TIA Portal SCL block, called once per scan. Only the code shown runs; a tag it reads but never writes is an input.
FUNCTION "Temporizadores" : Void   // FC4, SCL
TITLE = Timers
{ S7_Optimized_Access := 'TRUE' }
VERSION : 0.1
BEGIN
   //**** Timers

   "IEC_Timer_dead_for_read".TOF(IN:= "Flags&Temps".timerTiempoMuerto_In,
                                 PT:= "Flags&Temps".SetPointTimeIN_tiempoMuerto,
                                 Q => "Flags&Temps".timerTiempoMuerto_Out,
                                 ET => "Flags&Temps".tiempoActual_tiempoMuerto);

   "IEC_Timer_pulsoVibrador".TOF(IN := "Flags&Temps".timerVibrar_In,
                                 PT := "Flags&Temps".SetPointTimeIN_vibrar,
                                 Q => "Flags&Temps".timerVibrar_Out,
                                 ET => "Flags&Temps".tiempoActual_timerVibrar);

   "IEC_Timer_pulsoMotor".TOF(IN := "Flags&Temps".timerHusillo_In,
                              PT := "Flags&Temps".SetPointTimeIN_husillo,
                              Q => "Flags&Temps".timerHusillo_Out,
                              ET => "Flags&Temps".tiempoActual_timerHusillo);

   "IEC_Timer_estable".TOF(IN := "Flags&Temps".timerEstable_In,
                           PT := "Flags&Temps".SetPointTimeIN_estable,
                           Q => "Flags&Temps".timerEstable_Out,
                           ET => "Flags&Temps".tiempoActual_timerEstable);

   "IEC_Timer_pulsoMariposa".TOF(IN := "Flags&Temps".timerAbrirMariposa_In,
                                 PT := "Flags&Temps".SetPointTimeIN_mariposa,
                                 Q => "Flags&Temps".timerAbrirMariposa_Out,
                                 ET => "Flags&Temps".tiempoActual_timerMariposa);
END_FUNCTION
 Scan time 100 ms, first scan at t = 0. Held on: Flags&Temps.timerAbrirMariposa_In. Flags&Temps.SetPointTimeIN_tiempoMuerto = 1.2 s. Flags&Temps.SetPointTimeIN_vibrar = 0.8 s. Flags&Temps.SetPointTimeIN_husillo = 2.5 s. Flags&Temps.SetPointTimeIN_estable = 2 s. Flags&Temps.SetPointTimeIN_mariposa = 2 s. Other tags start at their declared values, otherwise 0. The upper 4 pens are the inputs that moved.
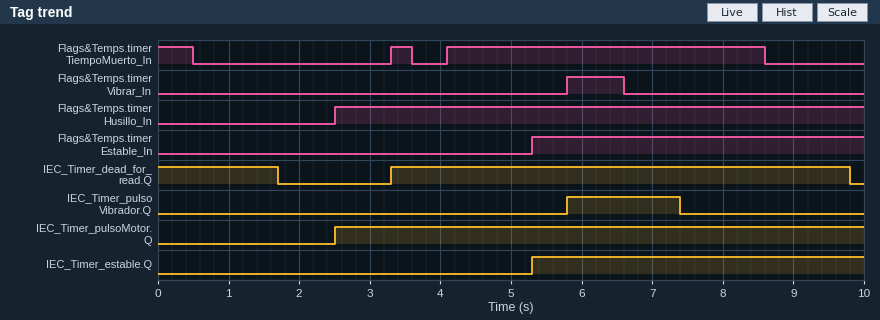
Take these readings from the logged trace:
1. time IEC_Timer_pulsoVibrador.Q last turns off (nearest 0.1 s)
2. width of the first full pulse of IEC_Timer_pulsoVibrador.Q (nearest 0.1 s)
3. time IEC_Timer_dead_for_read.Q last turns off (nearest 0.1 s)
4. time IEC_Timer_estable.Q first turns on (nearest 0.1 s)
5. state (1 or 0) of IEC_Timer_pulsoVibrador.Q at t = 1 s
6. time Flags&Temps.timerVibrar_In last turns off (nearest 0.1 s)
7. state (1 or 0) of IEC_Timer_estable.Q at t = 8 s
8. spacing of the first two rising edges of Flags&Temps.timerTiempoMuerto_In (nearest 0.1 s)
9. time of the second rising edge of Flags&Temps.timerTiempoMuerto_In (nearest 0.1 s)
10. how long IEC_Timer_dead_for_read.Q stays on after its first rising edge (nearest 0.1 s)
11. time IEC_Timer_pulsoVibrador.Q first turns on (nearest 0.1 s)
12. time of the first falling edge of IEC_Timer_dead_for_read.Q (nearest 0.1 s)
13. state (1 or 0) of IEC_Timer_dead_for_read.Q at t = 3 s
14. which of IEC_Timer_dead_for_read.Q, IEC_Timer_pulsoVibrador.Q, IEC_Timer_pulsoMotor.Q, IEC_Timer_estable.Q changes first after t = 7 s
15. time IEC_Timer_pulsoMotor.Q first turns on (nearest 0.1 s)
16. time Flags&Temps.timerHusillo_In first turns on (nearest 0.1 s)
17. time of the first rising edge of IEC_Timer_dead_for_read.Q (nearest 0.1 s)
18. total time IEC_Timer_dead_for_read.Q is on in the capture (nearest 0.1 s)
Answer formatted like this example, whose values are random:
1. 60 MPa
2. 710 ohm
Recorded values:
1. 7.4 s
2. 1.6 s
3. 9.8 s
4. 5.3 s
5. 0
6. 6.6 s
7. 1
8. 0.8 s
9. 4.1 s
10. 6.5 s
11. 5.8 s
12. 1.7 s
13. 0
14. IEC_Timer_pulsoVibrador.Q
15. 2.5 s
16. 2.5 s
17. 3.3 s
18. 8.2 s
